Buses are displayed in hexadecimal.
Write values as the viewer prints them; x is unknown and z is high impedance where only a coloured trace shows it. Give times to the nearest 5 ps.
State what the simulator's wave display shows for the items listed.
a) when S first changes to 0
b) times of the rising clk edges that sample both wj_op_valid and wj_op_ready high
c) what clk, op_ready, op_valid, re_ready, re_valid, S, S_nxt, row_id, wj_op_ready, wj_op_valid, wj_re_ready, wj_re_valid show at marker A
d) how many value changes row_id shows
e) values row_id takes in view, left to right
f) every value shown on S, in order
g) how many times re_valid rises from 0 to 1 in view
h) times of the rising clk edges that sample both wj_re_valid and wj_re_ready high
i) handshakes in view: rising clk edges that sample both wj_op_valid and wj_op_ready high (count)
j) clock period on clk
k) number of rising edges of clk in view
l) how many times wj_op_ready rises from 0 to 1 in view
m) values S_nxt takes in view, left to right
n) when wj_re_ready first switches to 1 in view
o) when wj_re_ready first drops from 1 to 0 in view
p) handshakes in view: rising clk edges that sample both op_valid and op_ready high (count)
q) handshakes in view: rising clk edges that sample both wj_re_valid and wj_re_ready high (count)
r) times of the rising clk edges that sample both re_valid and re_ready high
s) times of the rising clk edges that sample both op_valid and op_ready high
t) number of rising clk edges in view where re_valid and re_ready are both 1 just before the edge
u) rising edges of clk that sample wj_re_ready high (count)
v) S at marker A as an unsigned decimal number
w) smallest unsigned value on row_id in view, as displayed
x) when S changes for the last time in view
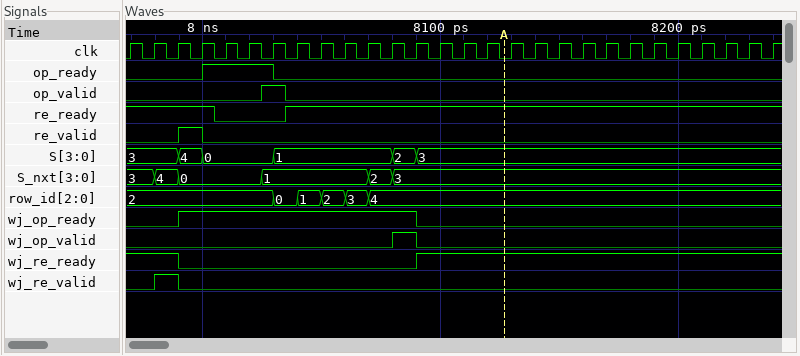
8000 ps
8090 ps
clk=0, op_ready=0, op_valid=0, re_ready=1, re_valid=0, S=3, S_nxt=3, row_id=4, wj_op_ready=0, wj_op_valid=0, wj_re_ready=1, wj_re_valid=0
5
2, 0, 1, 2, 3, 4
3, 4, 0, 1, 2, 3
1
7990 ps
1
10 ps
28
1
3, 4, 0, 1, 2, 3
8090 ps
7990 ps
1
1
8000 ps
8030 ps
1
18
3
0
8090 ps
